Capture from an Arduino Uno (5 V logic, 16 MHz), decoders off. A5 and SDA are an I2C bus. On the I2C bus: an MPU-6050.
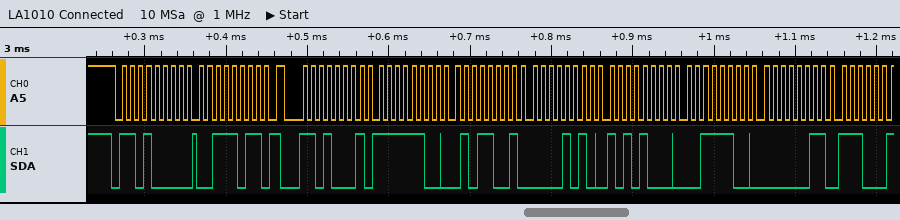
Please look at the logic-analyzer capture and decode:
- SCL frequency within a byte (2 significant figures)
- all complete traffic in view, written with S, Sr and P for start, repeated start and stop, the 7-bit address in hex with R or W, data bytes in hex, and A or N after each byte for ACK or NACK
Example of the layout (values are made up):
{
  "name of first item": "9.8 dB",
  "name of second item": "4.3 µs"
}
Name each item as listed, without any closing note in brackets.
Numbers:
{
  "SCL frequency within a byte": "100 kHz",
  "all complete traffic in view, written with S, Sr and P for start, repeated start and stop, the 7-bit address in hex with R or W, data bytes in hex, and A or N after each byte for ACK or NACK": "S 68W A 3B A Sr 68R A FC A 59 A 0A A A8 A 3C A 03 A"
}
